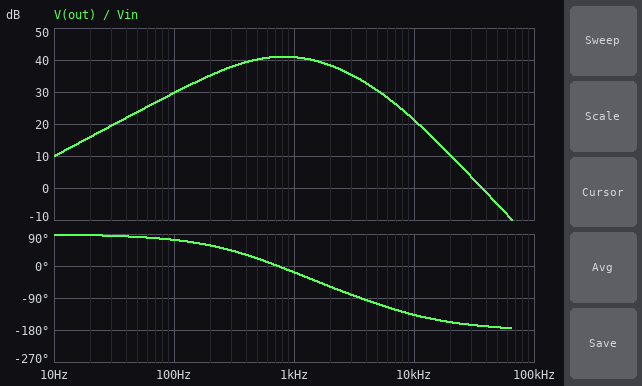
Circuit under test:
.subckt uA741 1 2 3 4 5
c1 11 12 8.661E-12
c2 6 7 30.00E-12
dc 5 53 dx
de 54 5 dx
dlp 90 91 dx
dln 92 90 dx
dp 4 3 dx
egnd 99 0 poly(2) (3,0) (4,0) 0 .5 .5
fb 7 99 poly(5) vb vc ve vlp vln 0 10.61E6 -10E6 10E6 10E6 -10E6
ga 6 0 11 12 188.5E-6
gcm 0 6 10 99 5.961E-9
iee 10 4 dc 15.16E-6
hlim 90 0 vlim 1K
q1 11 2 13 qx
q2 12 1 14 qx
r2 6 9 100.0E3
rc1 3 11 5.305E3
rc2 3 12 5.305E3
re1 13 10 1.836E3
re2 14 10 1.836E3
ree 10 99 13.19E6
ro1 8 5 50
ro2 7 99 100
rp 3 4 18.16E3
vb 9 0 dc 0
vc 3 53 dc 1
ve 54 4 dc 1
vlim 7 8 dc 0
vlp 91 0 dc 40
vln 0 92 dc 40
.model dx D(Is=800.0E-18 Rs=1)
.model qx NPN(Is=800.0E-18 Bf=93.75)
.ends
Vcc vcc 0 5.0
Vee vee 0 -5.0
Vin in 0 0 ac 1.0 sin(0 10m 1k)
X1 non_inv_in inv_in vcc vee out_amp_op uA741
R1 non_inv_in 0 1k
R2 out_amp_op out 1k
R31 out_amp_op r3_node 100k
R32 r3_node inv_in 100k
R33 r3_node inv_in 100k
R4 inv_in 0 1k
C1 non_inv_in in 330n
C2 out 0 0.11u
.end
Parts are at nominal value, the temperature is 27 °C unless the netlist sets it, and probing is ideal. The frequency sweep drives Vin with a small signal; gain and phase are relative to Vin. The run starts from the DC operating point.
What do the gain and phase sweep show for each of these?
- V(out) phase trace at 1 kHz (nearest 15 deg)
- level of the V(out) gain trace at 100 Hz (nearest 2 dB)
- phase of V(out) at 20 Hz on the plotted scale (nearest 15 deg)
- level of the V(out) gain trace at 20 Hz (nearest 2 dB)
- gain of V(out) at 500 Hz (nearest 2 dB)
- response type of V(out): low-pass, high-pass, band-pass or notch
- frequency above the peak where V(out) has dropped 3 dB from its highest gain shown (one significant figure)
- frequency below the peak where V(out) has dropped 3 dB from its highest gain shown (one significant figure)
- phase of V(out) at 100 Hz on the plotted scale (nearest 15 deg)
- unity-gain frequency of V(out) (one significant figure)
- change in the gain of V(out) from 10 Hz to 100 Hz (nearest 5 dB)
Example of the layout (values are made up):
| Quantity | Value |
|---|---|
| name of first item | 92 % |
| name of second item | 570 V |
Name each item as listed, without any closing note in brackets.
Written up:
| Quantity | Value |
|---|---|
| V(out) phase trace at 1 kHz | -15 deg |
| level of the V(out) gain trace at 100 Hz | 30 dB |
| phase of V(out) at 20 Hz on the plotted scale | 90 deg |
| level of the V(out) gain trace at 20 Hz | 16 dB |
| gain of V(out) at 500 Hz | 40 dB |
| response type of V(out): low-pass, high-pass, band-pass or notch | band-pass |
| frequency above the peak where V(out) has dropped 3 dB from its highest gain shown | 2 kHz |
| frequency below the peak where V(out) has dropped 3 dB from its highest gain shown | 300 Hz |
| phase of V(out) at 100 Hz on the plotted scale | 75 deg |
| unity-gain frequency of V(out) | 40 kHz |
| change in the gain of V(out) from 10 Hz to 100 Hz | 20 dB |
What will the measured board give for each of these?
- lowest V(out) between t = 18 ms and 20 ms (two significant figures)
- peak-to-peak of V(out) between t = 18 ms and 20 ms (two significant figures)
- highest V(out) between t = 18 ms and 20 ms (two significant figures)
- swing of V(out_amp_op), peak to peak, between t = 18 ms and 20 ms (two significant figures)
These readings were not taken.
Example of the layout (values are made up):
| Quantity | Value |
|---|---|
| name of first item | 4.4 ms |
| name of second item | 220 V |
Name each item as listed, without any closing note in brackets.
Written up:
| Quantity | Value |
|---|---|
| lowest V(out) between t = 18 ms and 20 ms | -1.1 V |
| peak-to-peak of V(out) between t = 18 ms and 20 ms | 2.2 V |
| highest V(out) between t = 18 ms and 20 ms | 1.1 V |
| swing of V(out_amp_op), peak to peak, between t = 18 ms and 20 ms | 2.7 V |
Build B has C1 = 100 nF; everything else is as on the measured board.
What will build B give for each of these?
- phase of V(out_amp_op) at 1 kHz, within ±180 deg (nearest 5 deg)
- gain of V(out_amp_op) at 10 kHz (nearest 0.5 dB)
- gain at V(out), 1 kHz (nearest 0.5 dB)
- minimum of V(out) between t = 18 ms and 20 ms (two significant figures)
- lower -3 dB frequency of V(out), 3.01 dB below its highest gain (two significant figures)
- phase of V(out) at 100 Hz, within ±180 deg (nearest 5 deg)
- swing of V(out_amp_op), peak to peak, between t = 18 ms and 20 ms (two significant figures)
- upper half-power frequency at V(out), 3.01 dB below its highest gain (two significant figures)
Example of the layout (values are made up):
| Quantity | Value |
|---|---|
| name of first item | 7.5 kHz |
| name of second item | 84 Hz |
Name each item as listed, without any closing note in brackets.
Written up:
| Quantity | Value |
|---|---|
| phase of V(out_amp_op) at 1 kHz, within ±180 deg | 50 deg |
| gain of V(out_amp_op) at 10 kHz | 38.0 dB |
| gain at V(out), 1 kHz | 36.5 dB |
| minimum of V(out) between t = 18 ms and 20 ms | -650 mV |
| lower -3 dB frequency of V(out), 3.01 dB below its highest gain | 610 Hz |
| phase of V(out) at 100 Hz, within ±180 deg | 80 deg |
| swing of V(out_amp_op), peak to peak, between t = 18 ms and 20 ms | 1.6 V |
| upper half-power frequency at V(out), 3.01 dB below its highest gain | 3.2 kHz |
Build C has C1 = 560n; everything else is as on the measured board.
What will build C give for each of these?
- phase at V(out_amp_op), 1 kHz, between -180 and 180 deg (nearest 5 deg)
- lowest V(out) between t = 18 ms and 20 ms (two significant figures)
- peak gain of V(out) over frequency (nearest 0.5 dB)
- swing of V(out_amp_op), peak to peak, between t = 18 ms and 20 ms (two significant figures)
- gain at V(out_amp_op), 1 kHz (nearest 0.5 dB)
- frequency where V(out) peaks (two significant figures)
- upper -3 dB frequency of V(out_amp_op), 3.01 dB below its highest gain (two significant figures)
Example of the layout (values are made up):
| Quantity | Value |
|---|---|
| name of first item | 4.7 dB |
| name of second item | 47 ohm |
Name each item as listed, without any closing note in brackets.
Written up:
| Quantity | Value |
|---|---|
| phase at V(out_amp_op), 1 kHz, between -180 and 180 deg | 5 deg |
| lowest V(out) between t = 18 ms and 20 ms | -1.2 V |
| peak gain of V(out) over frequency | 42.0 dB |
| swing of V(out_amp_op), peak to peak, between t = 18 ms and 20 ms | 2.9 V |
| gain at V(out_amp_op), 1 kHz | 43.0 dB |
| frequency where V(out) peaks | 630 Hz |
| upper -3 dB frequency of V(out_amp_op), 3.01 dB below its highest gain | 6.9 kHz |
